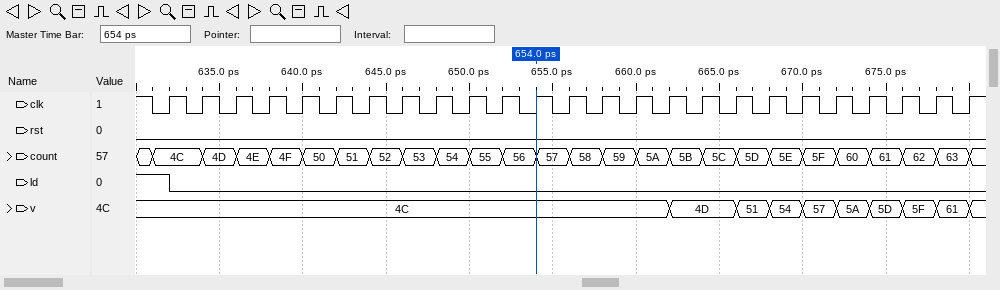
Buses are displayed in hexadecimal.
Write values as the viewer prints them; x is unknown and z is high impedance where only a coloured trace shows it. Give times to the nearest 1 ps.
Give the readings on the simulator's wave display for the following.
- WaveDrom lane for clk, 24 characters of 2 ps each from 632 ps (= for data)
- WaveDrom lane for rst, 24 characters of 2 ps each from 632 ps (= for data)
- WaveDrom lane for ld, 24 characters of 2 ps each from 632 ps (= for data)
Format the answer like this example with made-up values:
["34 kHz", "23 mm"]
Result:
["{name: 'clk', wave: 'p.......................'}", "{name: 'rst', wave: '0.......................'}", "{name: 'ld', wave: '0.......................'}"]
